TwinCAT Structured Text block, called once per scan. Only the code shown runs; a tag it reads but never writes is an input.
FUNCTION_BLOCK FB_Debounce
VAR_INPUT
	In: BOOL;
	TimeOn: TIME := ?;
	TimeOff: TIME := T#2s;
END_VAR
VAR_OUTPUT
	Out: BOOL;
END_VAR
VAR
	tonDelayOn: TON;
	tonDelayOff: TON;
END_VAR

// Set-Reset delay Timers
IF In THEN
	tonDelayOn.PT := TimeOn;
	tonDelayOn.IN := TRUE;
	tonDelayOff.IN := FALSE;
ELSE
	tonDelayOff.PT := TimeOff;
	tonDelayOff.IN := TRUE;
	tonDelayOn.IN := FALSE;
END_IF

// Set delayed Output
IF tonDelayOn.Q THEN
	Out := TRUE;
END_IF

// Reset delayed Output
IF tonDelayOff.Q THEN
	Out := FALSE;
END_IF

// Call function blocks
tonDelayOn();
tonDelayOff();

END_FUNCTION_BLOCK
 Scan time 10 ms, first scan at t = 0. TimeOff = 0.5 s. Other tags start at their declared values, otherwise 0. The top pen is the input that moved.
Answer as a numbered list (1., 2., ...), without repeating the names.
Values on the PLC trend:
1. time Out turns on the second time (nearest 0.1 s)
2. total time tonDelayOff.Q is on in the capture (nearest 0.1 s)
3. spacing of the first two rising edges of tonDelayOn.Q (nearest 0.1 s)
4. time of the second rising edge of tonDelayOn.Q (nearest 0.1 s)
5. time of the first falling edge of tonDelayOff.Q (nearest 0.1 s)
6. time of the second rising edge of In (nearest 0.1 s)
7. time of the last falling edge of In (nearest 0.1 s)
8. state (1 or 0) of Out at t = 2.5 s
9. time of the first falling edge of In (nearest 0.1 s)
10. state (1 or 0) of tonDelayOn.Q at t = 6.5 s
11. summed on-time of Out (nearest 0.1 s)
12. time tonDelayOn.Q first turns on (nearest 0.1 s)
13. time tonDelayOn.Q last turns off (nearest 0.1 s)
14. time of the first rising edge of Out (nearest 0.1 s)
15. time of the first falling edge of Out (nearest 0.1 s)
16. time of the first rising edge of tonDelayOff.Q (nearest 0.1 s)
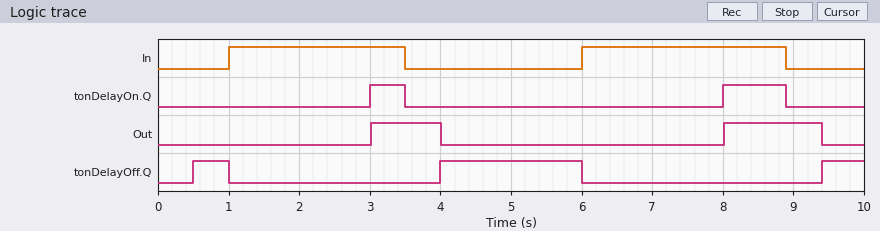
1. 8.0 s
2. 3.1 s
3. 5.0 s
4. 8.0 s
5. 1.0 s
6. 6.0 s
7. 8.9 s
8. 0
9. 3.5 s
10. 0
11. 2.4 s
12. 3.0 s
13. 8.9 s
14. 3.0 s
15. 4.0 s
16. 0.5 s
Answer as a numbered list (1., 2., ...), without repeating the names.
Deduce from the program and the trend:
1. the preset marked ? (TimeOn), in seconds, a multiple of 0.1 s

1. 2.0 s
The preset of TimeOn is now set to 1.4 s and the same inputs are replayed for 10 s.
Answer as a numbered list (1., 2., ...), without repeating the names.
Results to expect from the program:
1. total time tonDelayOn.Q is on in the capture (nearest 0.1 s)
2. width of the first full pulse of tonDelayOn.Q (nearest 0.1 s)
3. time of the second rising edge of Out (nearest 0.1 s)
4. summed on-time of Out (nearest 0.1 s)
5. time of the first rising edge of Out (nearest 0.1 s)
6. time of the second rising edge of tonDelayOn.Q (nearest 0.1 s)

1. 2.6 s
2. 1.1 s
3. 7.4 s
4. 3.6 s
5. 2.4 s
6. 7.4 s
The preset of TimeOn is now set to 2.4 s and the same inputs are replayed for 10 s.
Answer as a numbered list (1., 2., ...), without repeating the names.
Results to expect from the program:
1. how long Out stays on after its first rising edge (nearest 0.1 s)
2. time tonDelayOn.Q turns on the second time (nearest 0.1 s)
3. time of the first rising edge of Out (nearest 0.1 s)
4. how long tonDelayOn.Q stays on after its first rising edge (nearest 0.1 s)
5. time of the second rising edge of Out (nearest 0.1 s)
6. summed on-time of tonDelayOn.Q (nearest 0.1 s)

1. 0.6 s
2. 8.4 s
3. 3.4 s
4. 0.1 s
5. 8.4 s
6. 0.6 s
